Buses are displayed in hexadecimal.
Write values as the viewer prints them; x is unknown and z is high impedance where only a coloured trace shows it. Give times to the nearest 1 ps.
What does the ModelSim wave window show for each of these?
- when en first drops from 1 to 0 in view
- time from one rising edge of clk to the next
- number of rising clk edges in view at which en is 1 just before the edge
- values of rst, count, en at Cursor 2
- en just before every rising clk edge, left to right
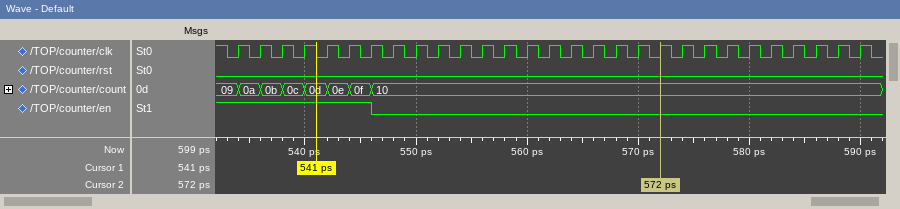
546 ps
2 ps
7
rst=0, count=10, en=0
1 1 1 1 1 1 1 0 0 0 0 0 0 0 0 0 0 0 0 0 0 0 0 0 0 0 0 0 0
